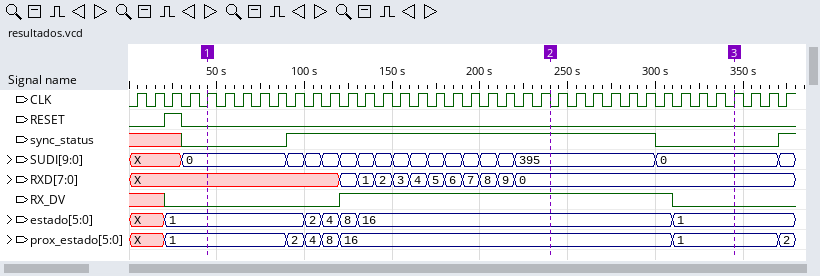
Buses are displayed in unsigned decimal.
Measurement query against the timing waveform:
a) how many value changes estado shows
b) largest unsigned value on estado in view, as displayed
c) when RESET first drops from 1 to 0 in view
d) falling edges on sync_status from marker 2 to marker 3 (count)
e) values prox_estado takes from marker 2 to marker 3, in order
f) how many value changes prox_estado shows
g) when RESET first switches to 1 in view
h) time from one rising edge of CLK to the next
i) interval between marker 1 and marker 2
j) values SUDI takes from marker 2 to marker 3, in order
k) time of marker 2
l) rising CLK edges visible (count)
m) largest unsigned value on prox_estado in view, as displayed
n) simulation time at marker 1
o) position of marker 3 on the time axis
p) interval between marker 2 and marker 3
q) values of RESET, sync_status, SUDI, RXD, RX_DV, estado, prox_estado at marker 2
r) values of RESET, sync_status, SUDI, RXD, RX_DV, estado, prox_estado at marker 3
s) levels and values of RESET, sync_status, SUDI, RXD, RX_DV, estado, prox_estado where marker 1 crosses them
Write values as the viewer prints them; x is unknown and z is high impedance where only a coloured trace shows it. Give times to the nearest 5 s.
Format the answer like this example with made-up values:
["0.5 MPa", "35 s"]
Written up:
["6", "16", "30 s", "1", "16, 1", "7", "20 s", "10 s", "195 s", "395, 0", "240 s", "38", "16", "45 s", "345 s", "105 s", "RESET=0, sync_status=1, SUDI=395, RXD=0, RX_DV=1, estado=16, prox_estado=16", "RESET=0, sync_status=0, SUDI=0, RXD=0, RX_DV=0, estado=1, prox_estado=1", "RESET=0, sync_status=0, SUDI=0, RXD=X, RX_DV=0, estado=1, prox_estado=1"]
